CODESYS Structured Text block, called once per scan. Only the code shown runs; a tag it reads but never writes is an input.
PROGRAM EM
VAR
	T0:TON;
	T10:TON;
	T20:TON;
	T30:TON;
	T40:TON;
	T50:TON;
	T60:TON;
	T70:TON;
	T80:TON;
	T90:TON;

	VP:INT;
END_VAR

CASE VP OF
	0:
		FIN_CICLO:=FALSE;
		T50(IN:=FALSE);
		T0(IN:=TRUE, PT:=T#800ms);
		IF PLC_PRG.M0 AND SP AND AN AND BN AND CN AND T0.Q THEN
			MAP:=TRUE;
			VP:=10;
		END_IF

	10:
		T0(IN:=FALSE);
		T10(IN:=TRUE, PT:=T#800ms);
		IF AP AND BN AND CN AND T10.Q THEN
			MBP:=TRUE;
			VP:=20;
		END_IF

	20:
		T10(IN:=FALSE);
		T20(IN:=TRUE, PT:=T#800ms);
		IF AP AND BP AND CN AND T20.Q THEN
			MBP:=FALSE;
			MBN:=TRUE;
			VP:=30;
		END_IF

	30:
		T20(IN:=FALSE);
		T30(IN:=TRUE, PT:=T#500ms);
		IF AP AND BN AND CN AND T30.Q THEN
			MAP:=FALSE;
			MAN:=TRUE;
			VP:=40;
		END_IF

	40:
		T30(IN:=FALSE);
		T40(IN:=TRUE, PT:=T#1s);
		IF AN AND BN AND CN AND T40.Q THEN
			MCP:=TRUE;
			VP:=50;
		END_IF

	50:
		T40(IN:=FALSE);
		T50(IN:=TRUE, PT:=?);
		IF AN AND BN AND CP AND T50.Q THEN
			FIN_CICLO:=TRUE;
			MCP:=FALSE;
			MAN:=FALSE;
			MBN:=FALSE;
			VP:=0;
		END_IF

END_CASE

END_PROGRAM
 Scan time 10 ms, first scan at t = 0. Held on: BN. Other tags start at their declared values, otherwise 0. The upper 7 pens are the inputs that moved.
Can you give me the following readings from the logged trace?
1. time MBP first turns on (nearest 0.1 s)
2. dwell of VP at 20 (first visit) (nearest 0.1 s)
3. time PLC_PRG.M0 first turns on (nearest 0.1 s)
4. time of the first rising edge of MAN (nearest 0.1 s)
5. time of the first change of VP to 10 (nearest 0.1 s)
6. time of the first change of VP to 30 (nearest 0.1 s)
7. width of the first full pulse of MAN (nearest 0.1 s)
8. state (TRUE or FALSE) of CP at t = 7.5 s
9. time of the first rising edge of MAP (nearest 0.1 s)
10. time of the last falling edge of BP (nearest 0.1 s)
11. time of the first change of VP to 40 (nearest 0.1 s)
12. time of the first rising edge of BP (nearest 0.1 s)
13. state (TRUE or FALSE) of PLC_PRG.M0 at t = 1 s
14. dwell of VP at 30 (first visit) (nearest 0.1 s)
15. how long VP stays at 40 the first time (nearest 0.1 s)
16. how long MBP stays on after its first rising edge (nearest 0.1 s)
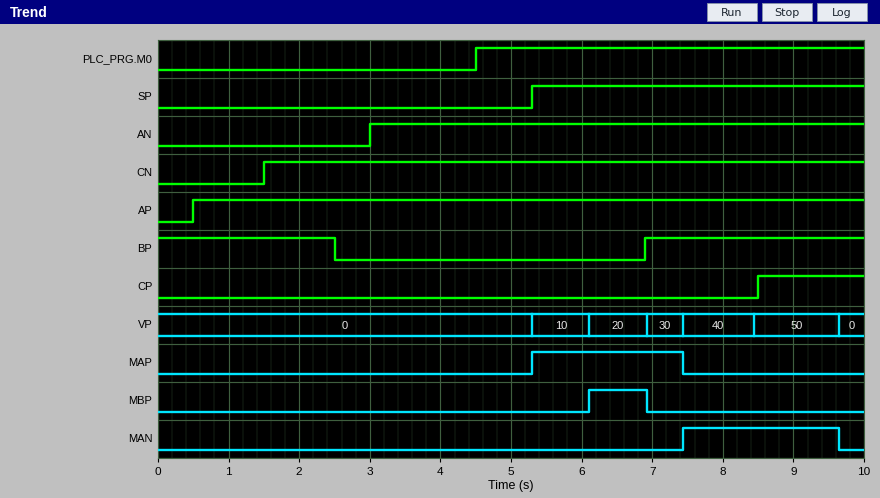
6.1 s
0.8 s
4.5 s
7.4 s
5.3 s
6.9 s
2.2 s
FALSE
5.3 s
2.5 s
7.4 s
6.9 s
FALSE
0.5 s
1.0 s
0.8 s
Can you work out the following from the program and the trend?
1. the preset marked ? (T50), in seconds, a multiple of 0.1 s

1.2 s
